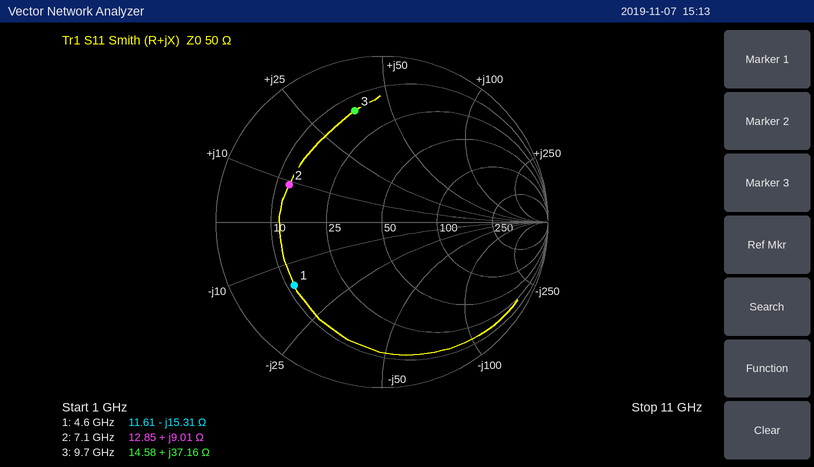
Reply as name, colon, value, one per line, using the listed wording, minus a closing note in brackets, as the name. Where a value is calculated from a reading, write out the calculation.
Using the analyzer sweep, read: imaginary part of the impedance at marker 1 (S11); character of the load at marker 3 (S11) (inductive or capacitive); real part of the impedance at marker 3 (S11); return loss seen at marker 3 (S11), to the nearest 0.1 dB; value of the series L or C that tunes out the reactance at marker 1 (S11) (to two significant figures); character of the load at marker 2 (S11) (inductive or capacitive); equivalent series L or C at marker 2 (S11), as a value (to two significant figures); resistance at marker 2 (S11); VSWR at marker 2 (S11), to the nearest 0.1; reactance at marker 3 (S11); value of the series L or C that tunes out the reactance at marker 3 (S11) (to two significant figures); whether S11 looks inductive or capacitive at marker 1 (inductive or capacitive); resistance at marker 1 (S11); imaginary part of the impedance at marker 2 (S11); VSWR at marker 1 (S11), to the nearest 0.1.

imaginary part of the impedance at marker 1: -15.31 Ω
character of the load at marker 3 (S11): inductive
real part of the impedance at marker 3: 14.58 Ω
return loss seen at marker 3 (S11), to the nearest 0.1 dB: 3.2 dB
value of the series L or C that tunes out the reactance at marker 1 (S11): L = 15.31 Ω/(2π × 4.6 GHz) ≈ 530 pH
character of the load at marker 2 (S11): inductive
equivalent series L or C at marker 2 (S11), as a value: L = 9.01 Ω/(2π × 7.1 GHz) ≈ 202 pH, so 200 pH to two significant figures
resistance at marker 2: 12.85 Ω
VSWR at marker 2 (S11), to the nearest 0.1: 4.0
reactance at marker 3: +37.16 Ω
value of the series L or C that tunes out the reactance at marker 3 (S11): C = 1/(2π × 9.7 GHz × 37.16 Ω) ≈ 442 fF, so 440 fF to two significant figures
whether S11 looks inductive or capacitive at marker 1: capacitive
resistance at marker 1: 11.61 Ω
imaginary part of the impedance at marker 2: +9.01 Ω
VSWR at marker 1 (S11), to the nearest 0.1: 4.7
